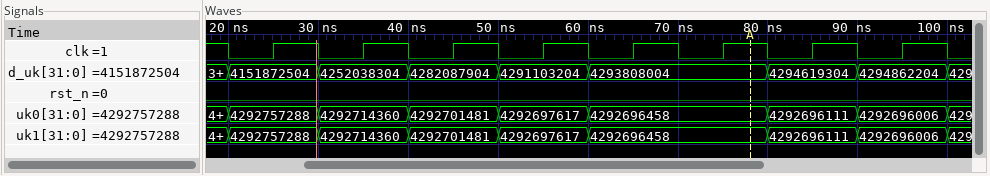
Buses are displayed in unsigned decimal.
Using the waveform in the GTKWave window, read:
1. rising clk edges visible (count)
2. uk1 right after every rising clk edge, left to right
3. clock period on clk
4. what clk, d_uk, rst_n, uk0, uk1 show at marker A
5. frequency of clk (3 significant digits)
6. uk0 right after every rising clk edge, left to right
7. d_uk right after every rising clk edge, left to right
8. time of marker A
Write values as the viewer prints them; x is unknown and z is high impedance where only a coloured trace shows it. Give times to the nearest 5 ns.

8
4292757288, 4292714360, 4292701481, 4292697617, 4292696458, 4292696458, 4292696111, 4292696006
10 ns
clk=1, d_uk=4293808004, rst_n=0, uk0=4292696458, uk1=4292696458
100 MHz
4292757288, 4292714360, 4292701481, 4292697617, 4292696458, 4292696458, 4292696111, 4292696006
4151872504, 4252038304, 4282087904, 4291103204, 4293808004, 4293808004, 4294619304, 4294862204
80 ns
